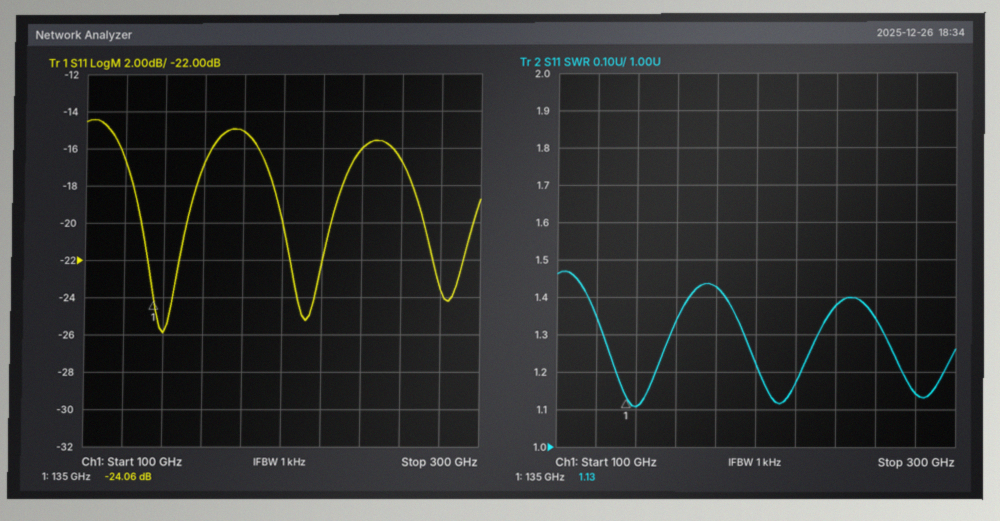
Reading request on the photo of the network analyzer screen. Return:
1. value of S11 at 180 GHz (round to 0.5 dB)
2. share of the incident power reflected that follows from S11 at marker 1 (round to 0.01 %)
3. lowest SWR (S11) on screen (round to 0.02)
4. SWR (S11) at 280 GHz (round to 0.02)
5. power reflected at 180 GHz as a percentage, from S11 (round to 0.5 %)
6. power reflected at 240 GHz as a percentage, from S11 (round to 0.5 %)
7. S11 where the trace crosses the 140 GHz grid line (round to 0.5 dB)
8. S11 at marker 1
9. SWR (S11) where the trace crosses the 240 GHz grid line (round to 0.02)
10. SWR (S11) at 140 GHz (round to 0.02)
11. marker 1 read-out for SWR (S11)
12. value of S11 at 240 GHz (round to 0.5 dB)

-15.0 dB
0.39 %
1.10
1.14
3.0 %
2.5 %
-26.0 dB
-24.06 dB
1.38
1.10
1.13
-16.0 dB
